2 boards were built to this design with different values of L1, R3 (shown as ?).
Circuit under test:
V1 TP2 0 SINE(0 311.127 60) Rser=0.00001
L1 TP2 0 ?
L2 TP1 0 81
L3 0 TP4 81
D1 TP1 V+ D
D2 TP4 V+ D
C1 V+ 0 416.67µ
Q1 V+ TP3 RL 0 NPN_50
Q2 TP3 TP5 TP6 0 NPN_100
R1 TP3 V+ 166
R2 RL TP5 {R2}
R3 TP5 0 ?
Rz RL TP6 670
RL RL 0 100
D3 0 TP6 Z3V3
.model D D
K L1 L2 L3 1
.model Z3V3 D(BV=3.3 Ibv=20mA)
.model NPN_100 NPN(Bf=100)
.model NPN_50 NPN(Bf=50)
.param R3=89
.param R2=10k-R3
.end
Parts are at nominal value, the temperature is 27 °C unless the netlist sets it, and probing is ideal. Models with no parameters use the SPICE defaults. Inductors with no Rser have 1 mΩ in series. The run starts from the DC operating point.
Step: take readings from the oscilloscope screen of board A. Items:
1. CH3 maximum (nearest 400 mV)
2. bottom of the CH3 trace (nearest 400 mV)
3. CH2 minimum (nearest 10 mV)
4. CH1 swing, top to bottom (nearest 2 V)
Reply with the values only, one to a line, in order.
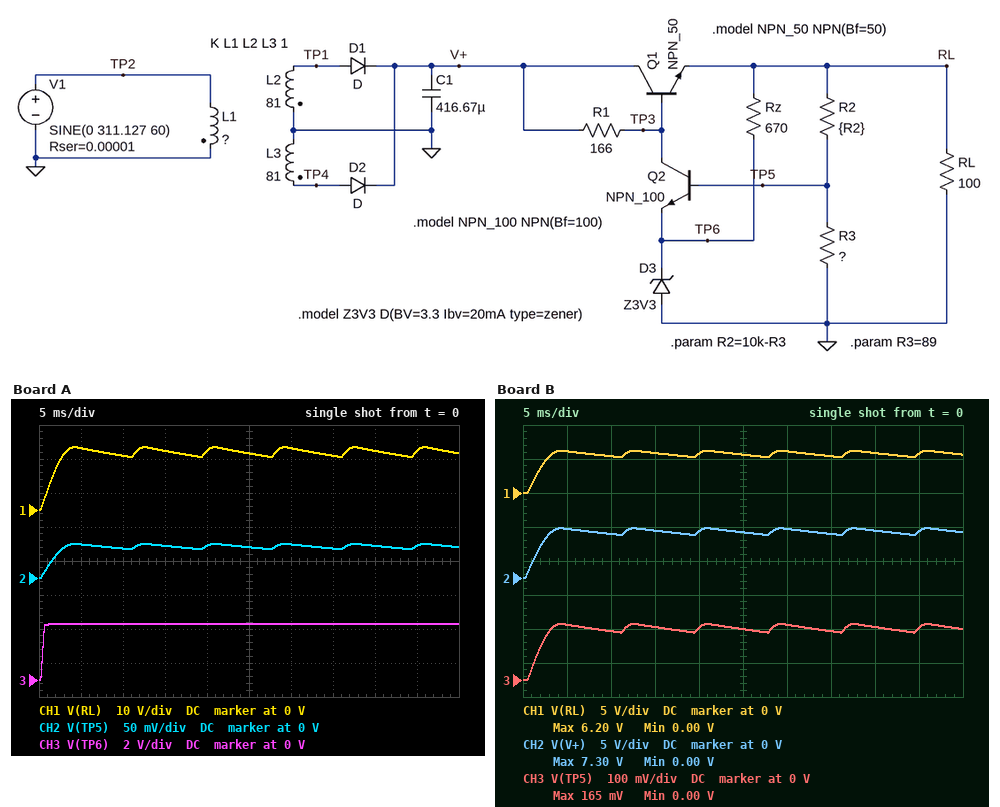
3.2 V
0 V
0 V
18 V
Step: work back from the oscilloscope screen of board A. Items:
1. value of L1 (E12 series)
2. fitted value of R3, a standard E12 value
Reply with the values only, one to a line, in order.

18 kH
27 Ω
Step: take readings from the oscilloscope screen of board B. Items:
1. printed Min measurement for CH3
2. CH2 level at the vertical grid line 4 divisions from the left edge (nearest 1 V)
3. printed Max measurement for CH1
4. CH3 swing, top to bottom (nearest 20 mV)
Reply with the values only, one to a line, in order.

0.00 V
7 V
6.20 V
160 mV
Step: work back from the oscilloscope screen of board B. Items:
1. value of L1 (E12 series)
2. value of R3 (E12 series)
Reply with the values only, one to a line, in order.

120 kH
270 Ω
